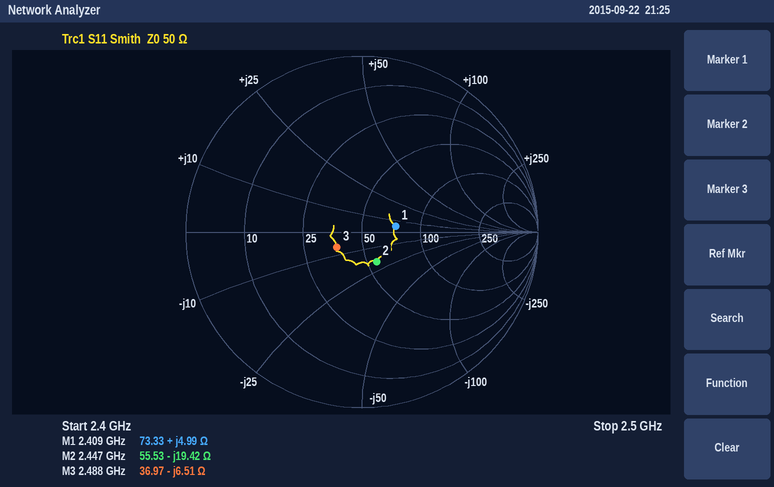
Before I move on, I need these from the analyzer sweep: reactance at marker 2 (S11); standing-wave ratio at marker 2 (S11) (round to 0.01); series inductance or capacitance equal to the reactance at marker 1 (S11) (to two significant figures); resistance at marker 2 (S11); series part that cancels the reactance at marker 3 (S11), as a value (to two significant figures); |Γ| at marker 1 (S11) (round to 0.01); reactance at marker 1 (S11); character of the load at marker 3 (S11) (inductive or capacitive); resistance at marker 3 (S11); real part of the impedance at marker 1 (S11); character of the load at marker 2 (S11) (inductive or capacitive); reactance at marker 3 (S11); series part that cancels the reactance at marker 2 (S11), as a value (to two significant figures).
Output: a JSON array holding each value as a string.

["-19.42 Ω", "1.46", "330 pH", "55.53 Ω", "420 pH", "0.19", "+4.99 Ω", "capacitive", "36.97 Ω", "73.33 Ω", "capacitive", "-6.51 Ω", "1.3 nH"]
